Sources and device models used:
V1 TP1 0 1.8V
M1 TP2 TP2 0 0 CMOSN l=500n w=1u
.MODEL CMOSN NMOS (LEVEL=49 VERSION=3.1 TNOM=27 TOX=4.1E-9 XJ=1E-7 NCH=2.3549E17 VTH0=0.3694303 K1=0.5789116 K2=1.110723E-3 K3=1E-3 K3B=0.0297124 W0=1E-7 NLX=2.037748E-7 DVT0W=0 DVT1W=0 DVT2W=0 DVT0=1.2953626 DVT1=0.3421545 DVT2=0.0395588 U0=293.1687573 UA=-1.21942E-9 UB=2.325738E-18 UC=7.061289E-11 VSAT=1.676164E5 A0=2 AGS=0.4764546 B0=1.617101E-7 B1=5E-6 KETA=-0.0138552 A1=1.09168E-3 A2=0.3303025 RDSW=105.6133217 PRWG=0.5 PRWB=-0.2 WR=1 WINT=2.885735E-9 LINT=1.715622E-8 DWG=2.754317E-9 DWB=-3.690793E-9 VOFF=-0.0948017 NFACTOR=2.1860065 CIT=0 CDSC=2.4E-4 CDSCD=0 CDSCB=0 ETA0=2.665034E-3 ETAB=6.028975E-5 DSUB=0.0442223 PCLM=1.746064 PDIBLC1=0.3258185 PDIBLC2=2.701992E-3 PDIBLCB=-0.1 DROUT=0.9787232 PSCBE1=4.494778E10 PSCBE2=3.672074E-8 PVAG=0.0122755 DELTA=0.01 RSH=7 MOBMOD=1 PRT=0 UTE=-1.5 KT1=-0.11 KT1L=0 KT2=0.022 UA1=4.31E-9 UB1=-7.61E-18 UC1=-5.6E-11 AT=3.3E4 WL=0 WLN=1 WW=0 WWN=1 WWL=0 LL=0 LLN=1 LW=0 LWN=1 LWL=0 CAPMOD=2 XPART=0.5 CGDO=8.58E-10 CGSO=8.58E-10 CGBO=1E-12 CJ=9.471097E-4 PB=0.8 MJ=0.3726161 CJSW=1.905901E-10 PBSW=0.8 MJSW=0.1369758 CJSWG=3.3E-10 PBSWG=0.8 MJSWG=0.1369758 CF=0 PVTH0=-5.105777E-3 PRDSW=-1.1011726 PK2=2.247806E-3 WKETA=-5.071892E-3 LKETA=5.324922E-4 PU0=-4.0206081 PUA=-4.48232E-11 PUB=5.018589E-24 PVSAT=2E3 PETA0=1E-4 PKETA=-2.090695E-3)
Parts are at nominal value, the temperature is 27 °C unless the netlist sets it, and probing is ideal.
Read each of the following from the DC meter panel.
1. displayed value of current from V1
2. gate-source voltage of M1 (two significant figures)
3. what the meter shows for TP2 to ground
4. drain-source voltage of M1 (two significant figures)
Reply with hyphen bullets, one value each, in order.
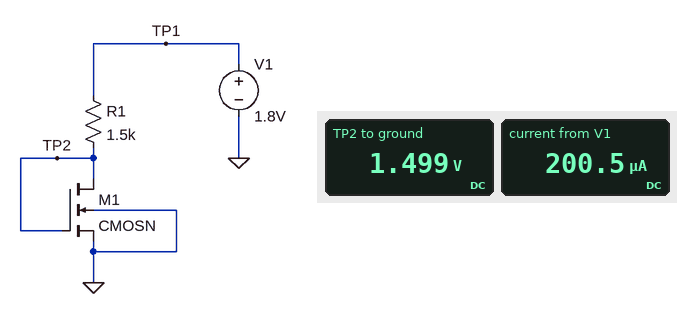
- 200.5 µA
- 1.5 V
- 1.499 V
- 1.5 V
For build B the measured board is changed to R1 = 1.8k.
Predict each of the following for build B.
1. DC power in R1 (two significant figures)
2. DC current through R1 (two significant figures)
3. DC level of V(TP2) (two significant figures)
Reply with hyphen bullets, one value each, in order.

- 64 µW
- 190 µA
- 1.5 V
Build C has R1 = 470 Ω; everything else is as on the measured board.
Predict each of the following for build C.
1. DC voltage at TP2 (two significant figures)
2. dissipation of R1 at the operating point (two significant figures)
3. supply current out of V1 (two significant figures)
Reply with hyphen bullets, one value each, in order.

- 1.7 V
- 30 µW
- 250 µA
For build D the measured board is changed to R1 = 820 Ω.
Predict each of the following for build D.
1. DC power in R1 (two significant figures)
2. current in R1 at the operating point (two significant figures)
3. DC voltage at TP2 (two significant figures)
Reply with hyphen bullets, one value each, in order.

- 44 µW
- 230 µA
- 1.6 V
